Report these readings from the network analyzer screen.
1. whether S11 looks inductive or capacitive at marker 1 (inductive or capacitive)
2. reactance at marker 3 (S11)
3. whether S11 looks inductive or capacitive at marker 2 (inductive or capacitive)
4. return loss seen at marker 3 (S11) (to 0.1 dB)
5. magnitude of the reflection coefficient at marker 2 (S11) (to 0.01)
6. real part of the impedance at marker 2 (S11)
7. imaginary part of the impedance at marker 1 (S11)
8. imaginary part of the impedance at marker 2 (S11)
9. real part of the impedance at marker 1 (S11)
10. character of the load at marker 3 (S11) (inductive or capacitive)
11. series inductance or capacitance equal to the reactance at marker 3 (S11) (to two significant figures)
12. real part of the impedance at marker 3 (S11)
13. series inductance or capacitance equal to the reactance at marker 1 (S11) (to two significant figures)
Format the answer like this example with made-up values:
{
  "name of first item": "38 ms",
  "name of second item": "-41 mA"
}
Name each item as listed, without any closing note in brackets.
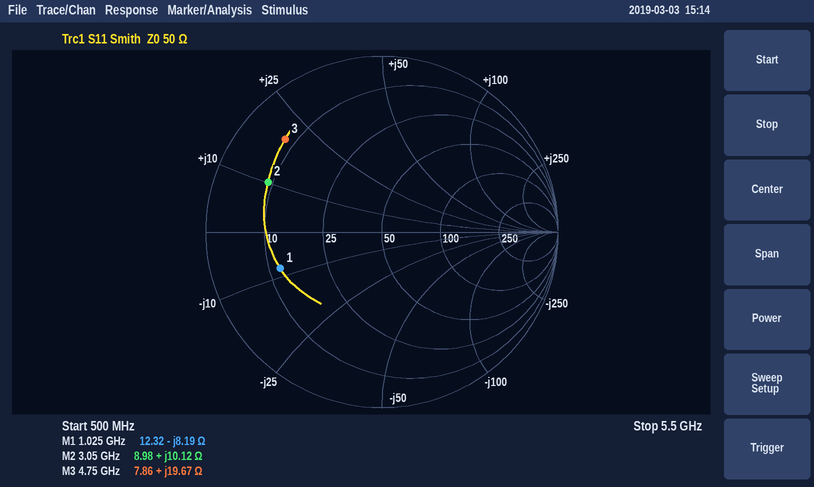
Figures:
{
  "whether S11 looks inductive or capacitive at marker 1": "capacitive",
  "reactance at marker 3": "+19.67 Ω",
  "whether S11 looks inductive or capacitive at marker 2": "inductive",
  "return loss seen at marker 3 (S11)": "2.4 dB",
  "magnitude of the reflection coefficient at marker 2 (S11)": "0.71",
  "real part of the impedance at marker 2": "8.98 Ω",
  "imaginary part of the impedance at marker 1": "-8.19 Ω",
  "imaginary part of the impedance at marker 2": "+10.12 Ω",
  "real part of the impedance at marker 1": "12.32 Ω",
  "character of the load at marker 3 (S11)": "inductive",
  "series inductance or capacitance equal to the reactance at marker 3 (S11)": "660 pH",
  "real part of the impedance at marker 3": "7.86 Ω",
  "series inductance or capacitance equal to the reactance at marker 1 (S11)": "19 pF"
}
